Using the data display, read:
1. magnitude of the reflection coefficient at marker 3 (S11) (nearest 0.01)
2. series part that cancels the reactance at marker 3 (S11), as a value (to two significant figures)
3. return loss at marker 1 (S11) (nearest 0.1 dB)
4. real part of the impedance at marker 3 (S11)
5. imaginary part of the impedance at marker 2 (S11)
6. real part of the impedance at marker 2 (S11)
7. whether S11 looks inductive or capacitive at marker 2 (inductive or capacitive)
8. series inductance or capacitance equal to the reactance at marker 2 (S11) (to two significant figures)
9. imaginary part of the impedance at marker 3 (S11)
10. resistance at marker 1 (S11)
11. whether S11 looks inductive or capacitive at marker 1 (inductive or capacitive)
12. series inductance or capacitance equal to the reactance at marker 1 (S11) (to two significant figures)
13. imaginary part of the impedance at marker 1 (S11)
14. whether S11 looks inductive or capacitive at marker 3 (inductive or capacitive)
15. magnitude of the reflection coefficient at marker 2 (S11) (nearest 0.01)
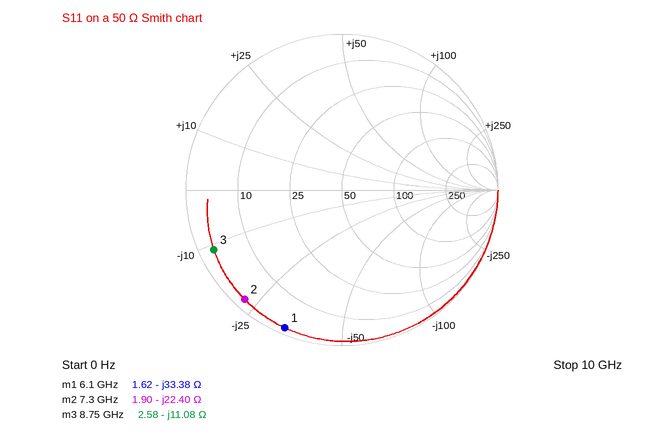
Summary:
0.91
200 pH
0.4 dB
2.58 Ω
-22.40 Ω
1.90 Ω
capacitive
970 fF
-11.08 Ω
1.62 Ω
capacitive
780 fF
-33.38 Ω
capacitive
0.94
